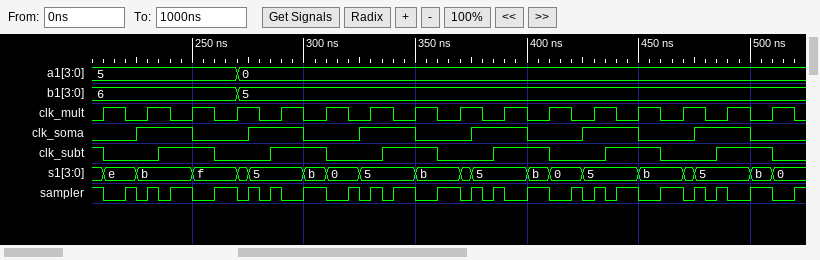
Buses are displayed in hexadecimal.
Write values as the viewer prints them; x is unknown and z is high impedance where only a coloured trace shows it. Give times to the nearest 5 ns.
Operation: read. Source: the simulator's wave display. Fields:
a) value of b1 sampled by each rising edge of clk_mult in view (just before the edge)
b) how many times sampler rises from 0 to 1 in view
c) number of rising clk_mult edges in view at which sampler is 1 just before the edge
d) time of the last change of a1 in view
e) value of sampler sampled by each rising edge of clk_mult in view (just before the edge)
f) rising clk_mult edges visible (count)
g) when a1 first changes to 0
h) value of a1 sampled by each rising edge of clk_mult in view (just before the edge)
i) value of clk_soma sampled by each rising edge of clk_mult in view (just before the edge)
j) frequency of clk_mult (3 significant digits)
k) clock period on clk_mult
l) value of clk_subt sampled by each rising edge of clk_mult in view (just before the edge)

6, 6, 6, 6, 5, 5, 5, 5, 5, 5, 5, 5, 5, 5, 5, 5
22
13
270 ns
1 0 1 1 1 1 0 1 1 1 1 0 1 1 1 1
16
270 ns
5, 5, 5, 5, 0, 0, 0, 0, 0, 0, 0, 0, 0, 0, 0, 0
0 1 1 0 1 0 1 1 0 1 0 1 1 0 1 0
50.0 MHz
20 ns
1 0 1 0 1 1 0 1 0 1 1 0 1 0 1 1
